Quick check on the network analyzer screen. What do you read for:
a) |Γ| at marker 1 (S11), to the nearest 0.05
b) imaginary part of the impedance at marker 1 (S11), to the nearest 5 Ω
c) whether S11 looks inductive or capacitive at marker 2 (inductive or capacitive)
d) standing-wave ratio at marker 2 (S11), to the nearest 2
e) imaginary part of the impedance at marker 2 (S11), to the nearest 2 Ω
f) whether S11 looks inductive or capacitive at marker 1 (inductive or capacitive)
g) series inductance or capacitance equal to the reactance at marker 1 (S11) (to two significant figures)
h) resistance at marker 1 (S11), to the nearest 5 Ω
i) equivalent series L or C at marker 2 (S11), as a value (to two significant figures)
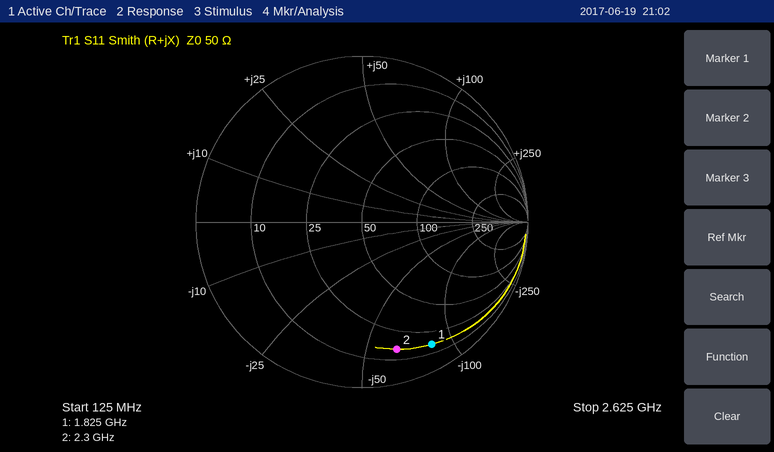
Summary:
0.85
-85 Ω
capacitive
8
-64 Ω
capacitive
1.0 pF
15 Ω
1.1 pF
